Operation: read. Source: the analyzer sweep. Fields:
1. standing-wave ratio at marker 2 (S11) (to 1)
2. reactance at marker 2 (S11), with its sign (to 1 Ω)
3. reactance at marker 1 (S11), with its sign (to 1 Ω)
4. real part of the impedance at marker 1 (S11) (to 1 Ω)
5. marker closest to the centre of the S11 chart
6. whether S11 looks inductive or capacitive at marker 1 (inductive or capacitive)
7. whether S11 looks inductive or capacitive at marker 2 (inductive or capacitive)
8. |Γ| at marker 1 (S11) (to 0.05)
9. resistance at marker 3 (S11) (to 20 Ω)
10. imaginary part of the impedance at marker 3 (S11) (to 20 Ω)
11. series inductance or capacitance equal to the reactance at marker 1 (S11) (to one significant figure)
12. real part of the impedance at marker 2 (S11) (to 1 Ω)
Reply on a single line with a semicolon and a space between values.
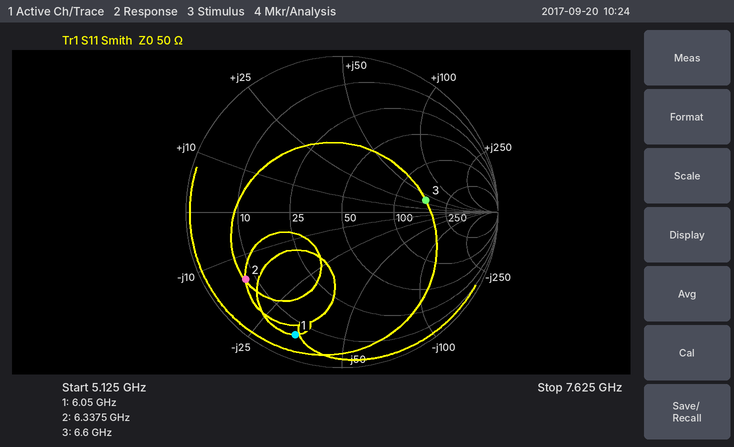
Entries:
7; -15 Ω; -34 Ω; 6 Ω; marker 3; capacitive; capacitive; 0.85; 160 Ω; +40 Ω; 800 fF; 8 Ω
